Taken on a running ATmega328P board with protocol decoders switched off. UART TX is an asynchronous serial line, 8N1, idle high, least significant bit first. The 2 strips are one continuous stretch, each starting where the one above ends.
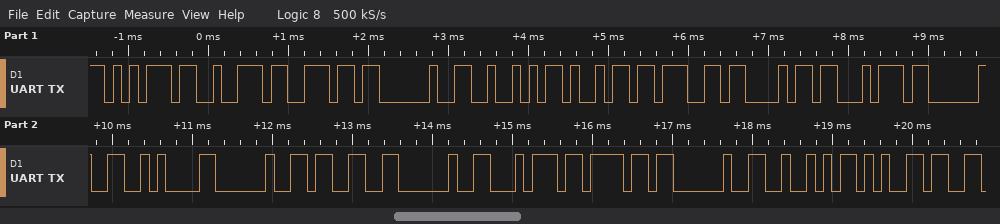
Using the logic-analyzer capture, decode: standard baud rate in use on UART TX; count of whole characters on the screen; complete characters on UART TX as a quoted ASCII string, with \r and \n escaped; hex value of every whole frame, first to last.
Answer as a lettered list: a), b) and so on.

a) 9600 baud
b) 19
c) "urn Right \n 3 to Re"
d) 75 72 6E 20 52 69 67 68 74 20 0A 20 33 20 74 6F 20 52 65
